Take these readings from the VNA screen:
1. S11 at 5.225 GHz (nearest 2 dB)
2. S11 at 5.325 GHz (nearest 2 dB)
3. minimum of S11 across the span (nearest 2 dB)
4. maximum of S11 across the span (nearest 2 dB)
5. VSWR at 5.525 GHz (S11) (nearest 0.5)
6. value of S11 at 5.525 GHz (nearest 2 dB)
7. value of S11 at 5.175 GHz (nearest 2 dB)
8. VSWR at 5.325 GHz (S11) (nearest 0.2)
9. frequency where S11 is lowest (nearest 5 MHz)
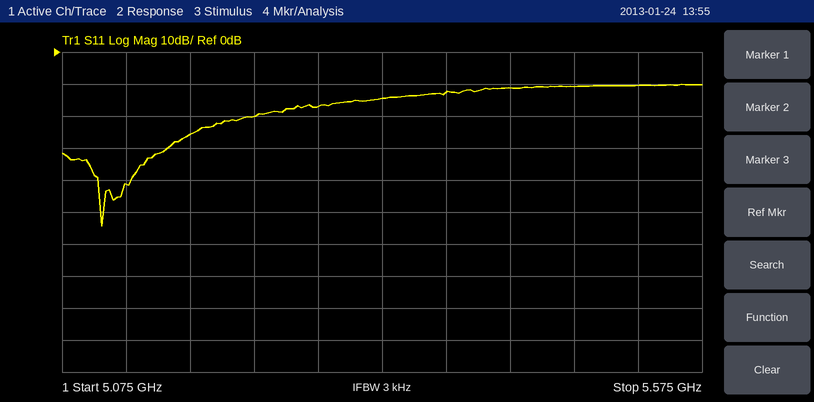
-20 dB
-14 dB
-54 dB
-10 dB
2.0
-10 dB
-26 dB
1.4
5.105 GHz
